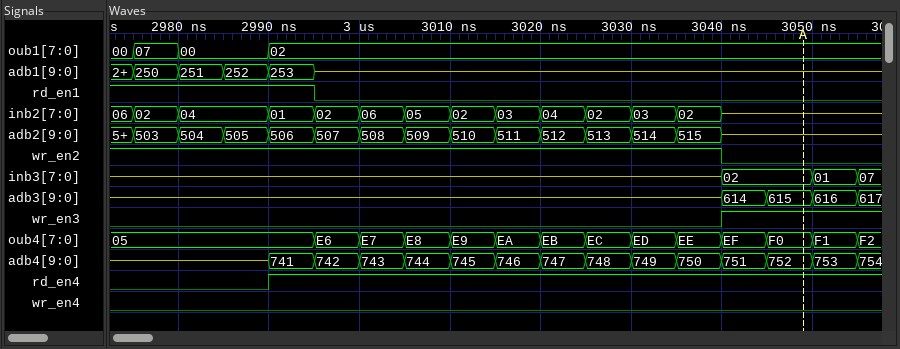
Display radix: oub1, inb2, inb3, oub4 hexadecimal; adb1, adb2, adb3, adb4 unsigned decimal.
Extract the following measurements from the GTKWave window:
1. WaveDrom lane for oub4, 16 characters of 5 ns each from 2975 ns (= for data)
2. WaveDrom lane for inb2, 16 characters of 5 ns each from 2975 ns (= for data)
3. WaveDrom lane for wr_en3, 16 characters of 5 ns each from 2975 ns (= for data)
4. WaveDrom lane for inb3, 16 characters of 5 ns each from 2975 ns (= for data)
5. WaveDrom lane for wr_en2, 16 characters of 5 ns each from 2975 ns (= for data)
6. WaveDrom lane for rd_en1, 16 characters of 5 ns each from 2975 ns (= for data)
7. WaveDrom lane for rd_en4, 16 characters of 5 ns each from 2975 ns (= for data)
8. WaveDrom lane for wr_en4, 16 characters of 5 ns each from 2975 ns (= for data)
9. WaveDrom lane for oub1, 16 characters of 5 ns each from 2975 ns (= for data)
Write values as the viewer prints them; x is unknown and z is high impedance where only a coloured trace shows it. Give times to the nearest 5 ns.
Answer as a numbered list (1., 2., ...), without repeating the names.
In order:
1. {name: 'oub4', wave: '=...============', data: '05 E6 E7 E8 E9 EA EB EC ED EE EF F0 F1'}
2. {name: 'inb2', wave: '==.==========z..', data: '02 04 01 02 06 05 02 03 04 02 03 02'}
3. {name: 'wr_en3', wave: '0............1..'}
4. {name: 'inb3', wave: 'z............=.=', data: '02 01'}
5. {name: 'wr_en2', wave: '1............0..'}
6. {name: 'rd_en1', wave: '1...0...........'}
7. {name: 'rd_en4', wave: '0..1............'}
8. {name: 'wr_en4', wave: '0...............'}
9. {name: 'oub1', wave: '==.=............', data: '07 00 02'}
